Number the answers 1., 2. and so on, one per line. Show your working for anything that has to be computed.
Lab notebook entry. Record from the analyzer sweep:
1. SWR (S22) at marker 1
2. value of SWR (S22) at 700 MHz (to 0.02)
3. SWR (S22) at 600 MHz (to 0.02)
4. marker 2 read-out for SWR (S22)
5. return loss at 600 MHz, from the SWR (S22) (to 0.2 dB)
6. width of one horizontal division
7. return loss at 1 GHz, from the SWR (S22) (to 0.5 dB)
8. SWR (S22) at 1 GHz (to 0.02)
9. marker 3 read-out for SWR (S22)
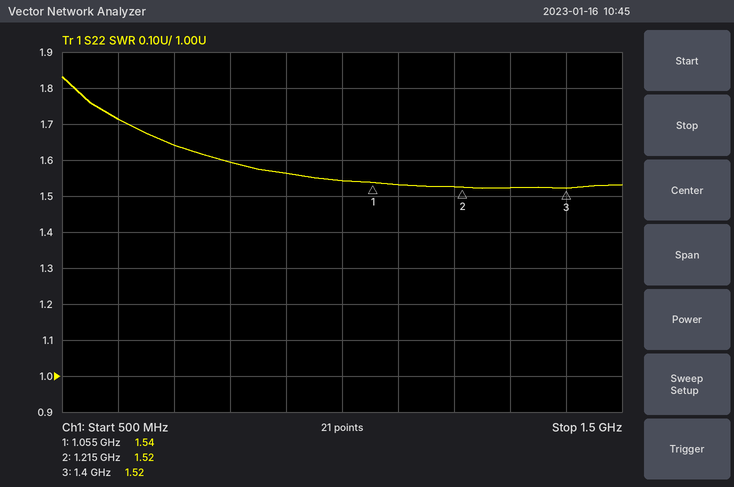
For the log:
1. 1.54
2. 1.64
3. 1.72
4. 1.52
5. −20 log10((1.72 − 1)/(1.72 + 1)) ≈ 11.5 dB, so 11.6 dB to the nearest 0.2 dB
6. 100 MHz
7. −20 log10((1.54 − 1)/(1.54 + 1)) ≈ 13.4 dB, so 13.5 dB to the nearest 0.5 dB
8. 1.54
9. 1.52
